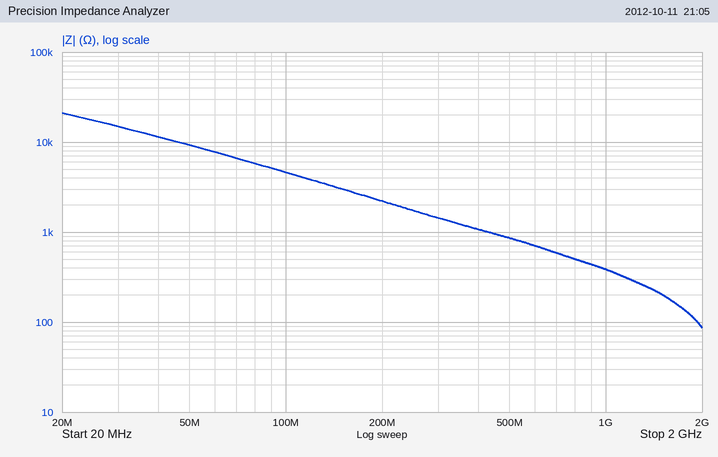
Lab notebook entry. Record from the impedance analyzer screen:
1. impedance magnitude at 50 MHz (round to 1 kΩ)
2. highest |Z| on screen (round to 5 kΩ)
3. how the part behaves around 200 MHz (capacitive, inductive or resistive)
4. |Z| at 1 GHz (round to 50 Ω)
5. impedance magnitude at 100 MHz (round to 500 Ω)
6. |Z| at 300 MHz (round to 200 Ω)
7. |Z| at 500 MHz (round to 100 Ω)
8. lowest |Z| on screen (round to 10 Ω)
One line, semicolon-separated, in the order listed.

9 kΩ; 20 kΩ; capacitive; 400 Ω; 4.5 kΩ; 1.4 kΩ; 900 Ω; 90 Ω
